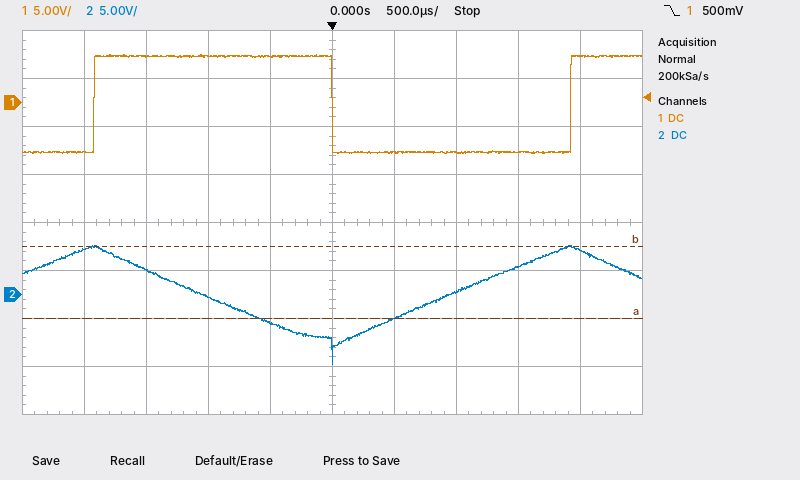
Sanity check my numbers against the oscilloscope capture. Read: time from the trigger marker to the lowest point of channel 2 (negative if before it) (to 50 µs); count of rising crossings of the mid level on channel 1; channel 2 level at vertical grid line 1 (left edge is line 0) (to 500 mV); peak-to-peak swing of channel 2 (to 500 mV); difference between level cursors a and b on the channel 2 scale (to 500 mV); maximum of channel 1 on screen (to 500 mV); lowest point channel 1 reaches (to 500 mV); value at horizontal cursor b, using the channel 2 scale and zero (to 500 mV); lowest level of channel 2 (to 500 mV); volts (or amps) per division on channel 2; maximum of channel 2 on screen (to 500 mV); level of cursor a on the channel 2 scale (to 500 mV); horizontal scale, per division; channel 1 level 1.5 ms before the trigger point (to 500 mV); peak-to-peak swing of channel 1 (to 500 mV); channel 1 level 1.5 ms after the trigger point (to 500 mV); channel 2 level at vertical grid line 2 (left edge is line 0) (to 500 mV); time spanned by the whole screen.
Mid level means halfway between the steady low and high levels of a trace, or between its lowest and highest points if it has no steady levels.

0 µs
2
4.5 V
12.5 V
7.5 V
5.0 V
-5.5 V
5.0 V
-7.5 V
5 V
5.0 V
-2.5 V
500 µs
5.0 V
10.5 V
-5.0 V
2.5 V
5 ms
